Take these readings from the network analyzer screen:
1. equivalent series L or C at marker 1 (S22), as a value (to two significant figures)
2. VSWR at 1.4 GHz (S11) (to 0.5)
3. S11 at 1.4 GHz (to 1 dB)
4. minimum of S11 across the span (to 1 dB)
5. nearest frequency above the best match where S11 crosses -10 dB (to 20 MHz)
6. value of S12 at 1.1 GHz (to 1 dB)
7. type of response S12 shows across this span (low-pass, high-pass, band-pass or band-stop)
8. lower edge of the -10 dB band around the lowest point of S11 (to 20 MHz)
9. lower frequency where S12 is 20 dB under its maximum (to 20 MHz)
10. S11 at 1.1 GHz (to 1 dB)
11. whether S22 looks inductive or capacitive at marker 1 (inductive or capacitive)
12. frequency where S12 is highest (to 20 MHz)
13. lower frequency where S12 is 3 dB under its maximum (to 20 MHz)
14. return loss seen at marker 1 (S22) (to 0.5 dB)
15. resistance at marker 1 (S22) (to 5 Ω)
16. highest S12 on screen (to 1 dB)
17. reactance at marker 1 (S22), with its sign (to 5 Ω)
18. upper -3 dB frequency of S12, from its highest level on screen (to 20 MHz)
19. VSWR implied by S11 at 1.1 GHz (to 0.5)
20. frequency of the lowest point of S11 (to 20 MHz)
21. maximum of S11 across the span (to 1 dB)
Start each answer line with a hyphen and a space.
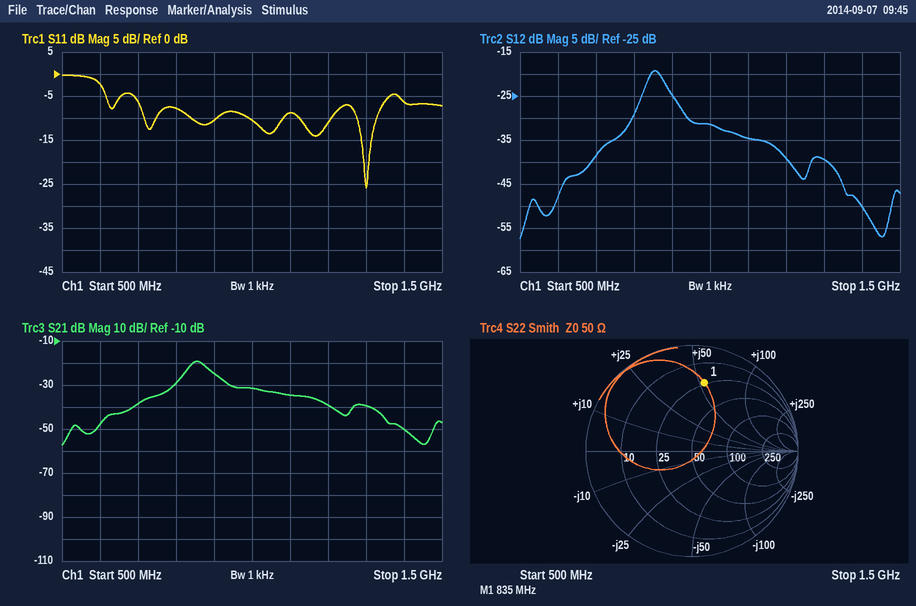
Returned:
- 10 nH
- 3.0
- -6 dB
- -26 dB
- 1.32 GHz
- -35 dB
- band-pass
- 1.28 GHz
- 700 MHz
- -9 dB
- inductive
- 860 MHz
- 840 MHz
- 3.5 dB
- 25 Ω
- -19 dB
- +55 Ω
- 880 MHz
- 2.0
- 1.30 GHz
- 0 dB
